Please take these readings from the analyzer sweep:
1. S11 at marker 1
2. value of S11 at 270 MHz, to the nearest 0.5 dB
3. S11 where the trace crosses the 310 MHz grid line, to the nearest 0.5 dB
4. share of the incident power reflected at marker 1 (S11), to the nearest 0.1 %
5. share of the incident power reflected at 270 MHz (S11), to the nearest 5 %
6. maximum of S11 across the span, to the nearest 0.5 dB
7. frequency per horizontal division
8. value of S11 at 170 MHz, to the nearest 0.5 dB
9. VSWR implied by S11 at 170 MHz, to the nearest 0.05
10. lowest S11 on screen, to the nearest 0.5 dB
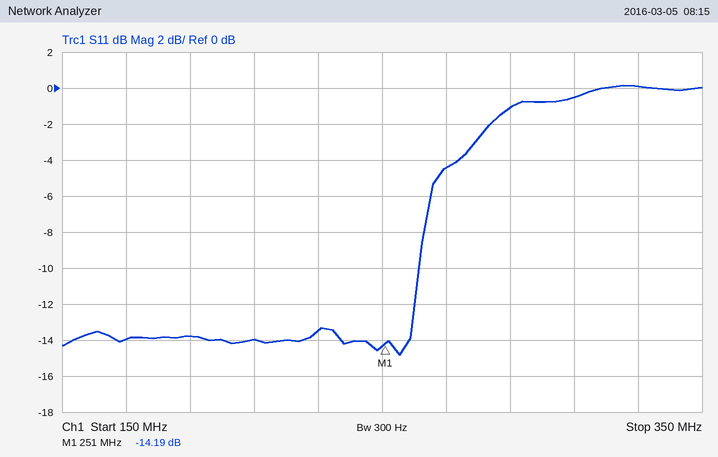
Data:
-14.19 dB
-4.5 dB
-0.5 dB
3.8 %
35 %
0.0 dB
20 MHz
-14.0 dB
1.50
-15.0 dB
